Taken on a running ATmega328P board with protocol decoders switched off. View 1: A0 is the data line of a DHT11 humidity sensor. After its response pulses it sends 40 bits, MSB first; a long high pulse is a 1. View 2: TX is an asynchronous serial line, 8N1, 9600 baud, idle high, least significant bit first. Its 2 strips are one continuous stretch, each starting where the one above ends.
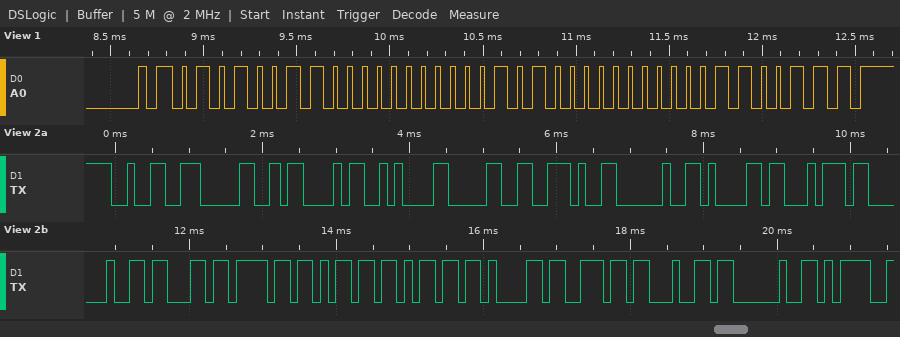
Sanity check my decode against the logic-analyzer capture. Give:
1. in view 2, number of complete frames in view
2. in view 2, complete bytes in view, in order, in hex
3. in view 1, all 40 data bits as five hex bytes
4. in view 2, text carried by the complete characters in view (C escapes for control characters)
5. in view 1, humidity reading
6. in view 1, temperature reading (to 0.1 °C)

19
32 30 43 0A 30 2E 20 61 74 20 63 6F 6D 6D 61 6E 64 20 3D
53 00 14 00 67
"20C\n0. at command ="
83 %
20.0 °C
